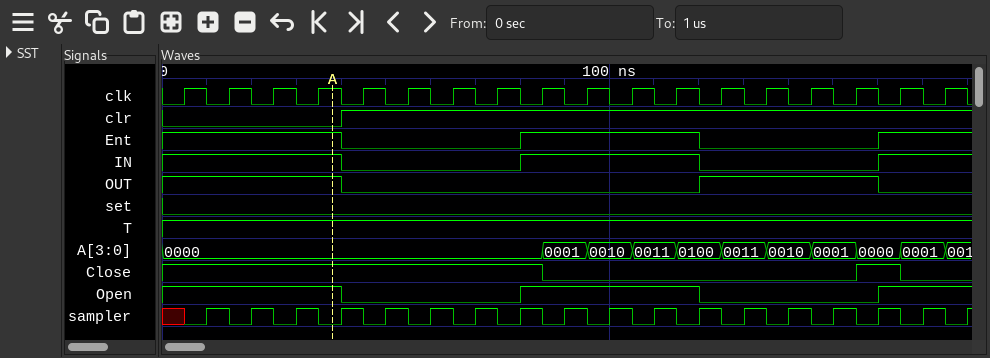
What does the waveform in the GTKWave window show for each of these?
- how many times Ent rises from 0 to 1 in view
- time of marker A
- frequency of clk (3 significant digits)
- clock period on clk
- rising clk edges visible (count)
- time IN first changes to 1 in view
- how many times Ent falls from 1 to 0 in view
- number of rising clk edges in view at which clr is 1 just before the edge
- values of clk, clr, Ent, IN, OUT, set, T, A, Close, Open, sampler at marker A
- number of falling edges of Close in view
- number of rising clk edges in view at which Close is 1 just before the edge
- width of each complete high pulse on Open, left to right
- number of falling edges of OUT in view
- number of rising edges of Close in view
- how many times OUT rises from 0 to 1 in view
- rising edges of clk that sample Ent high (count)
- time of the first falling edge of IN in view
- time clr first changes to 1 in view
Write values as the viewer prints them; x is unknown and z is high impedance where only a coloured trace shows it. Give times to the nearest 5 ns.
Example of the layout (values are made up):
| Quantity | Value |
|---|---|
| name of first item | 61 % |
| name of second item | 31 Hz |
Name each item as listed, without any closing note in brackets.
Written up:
| Quantity | Value |
|---|---|
| how many times Ent rises from 0 to 1 in view | 2 |
| time of marker A | 40 ns |
| frequency of clk | 100 MHz |
| clock period on clk | 10 ns |
| rising clk edges visible | 18 |
| time IN first changes to 1 in view | 80 ns |
| how many times Ent falls from 1 to 0 in view | 2 |
| number of rising clk edges in view at which clr is 1 just before the edge | 14 |
| values of clk, clr, Ent, IN, OUT, set, T, A, Close, Open, sampler at marker A | clk=1, clr=0, Ent=1, IN=1, OUT=1, set=0, T=1, A=0000, Close=1, Open=1, sampler=0 |
| number of falling edges of Close in view | 2 |
| number of rising clk edges in view at which Close is 1 just before the edge | 10 |
| width of each complete high pulse on Open, left to right | 40 ns |
| number of falling edges of OUT in view | 2 |
| number of rising edges of Close in view | 1 |
| how many times OUT rises from 0 to 1 in view | 1 |
| rising edges of clk that sample Ent high | 10 |
| time of the first falling edge of IN in view | 40 ns |
| time clr first changes to 1 in view | 40 ns |
